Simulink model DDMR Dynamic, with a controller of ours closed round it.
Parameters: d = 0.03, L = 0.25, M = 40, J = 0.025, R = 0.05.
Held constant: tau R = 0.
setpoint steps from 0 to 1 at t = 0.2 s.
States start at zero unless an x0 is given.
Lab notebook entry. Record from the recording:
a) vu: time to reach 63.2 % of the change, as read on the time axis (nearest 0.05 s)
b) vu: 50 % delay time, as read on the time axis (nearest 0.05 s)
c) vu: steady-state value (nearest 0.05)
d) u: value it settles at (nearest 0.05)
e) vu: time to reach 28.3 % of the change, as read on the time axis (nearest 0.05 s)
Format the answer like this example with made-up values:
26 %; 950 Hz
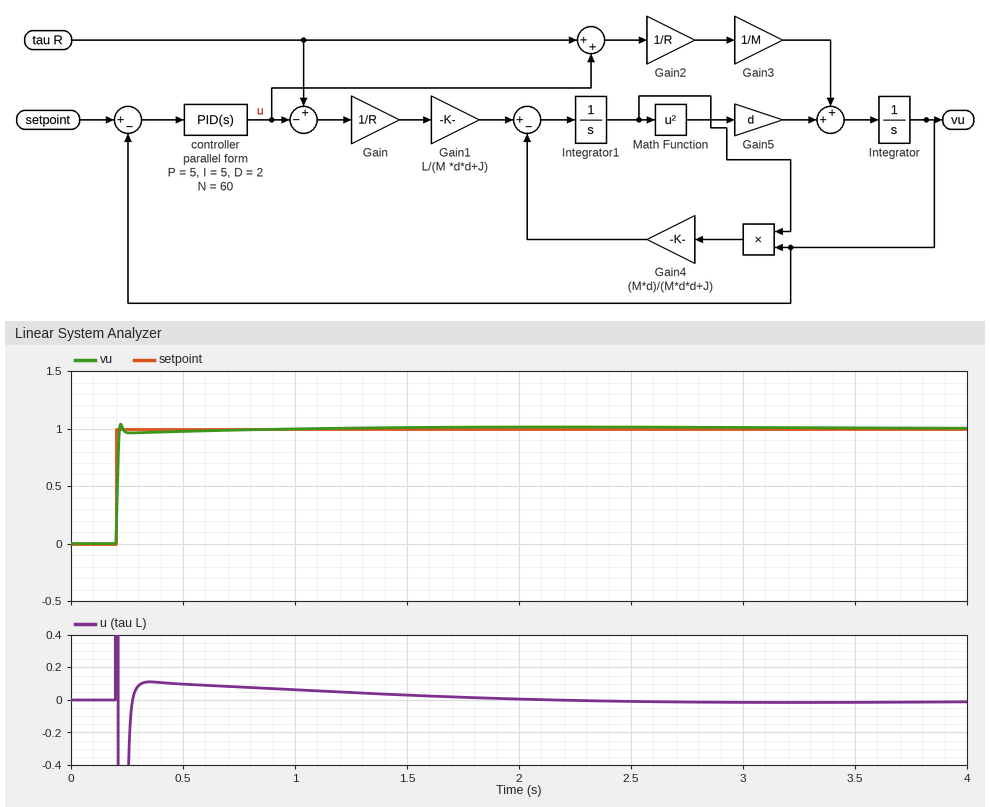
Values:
0.20 s; 0.20 s; 1.00; 0.00; 0.20 s
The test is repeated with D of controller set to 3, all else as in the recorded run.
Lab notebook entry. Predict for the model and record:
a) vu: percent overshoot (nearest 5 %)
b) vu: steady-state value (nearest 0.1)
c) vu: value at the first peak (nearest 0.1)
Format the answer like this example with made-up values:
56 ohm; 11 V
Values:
10 %; 1.0; 1.1
